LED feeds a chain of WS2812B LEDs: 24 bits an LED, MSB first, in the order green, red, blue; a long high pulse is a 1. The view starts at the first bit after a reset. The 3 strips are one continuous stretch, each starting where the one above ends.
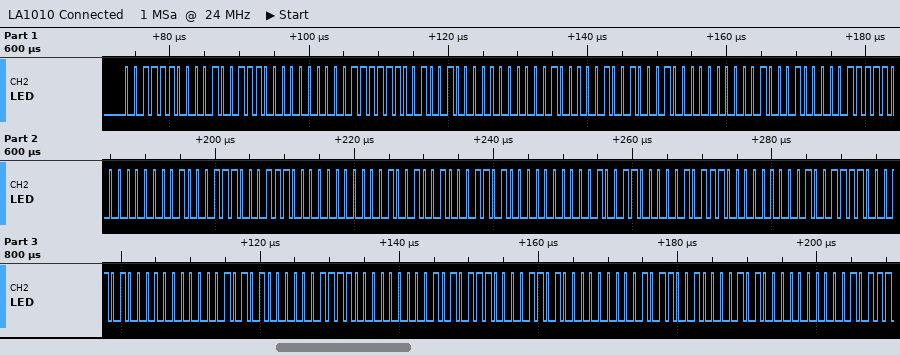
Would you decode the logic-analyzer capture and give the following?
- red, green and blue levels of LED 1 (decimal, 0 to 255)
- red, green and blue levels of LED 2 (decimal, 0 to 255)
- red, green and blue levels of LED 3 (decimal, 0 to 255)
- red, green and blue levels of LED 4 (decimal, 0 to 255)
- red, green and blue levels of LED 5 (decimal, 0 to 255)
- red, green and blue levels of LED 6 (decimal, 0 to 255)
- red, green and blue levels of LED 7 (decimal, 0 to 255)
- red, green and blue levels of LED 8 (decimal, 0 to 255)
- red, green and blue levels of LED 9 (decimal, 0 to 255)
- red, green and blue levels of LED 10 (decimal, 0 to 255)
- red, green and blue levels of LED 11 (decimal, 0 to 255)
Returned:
39, 60, 0
36, 63, 0
34, 65, 0
31, 68, 0
28, 71, 0
26, 73, 0
23, 76, 0
20, 79, 0
15, 84, 0
13, 87, 0
10, 89, 0
